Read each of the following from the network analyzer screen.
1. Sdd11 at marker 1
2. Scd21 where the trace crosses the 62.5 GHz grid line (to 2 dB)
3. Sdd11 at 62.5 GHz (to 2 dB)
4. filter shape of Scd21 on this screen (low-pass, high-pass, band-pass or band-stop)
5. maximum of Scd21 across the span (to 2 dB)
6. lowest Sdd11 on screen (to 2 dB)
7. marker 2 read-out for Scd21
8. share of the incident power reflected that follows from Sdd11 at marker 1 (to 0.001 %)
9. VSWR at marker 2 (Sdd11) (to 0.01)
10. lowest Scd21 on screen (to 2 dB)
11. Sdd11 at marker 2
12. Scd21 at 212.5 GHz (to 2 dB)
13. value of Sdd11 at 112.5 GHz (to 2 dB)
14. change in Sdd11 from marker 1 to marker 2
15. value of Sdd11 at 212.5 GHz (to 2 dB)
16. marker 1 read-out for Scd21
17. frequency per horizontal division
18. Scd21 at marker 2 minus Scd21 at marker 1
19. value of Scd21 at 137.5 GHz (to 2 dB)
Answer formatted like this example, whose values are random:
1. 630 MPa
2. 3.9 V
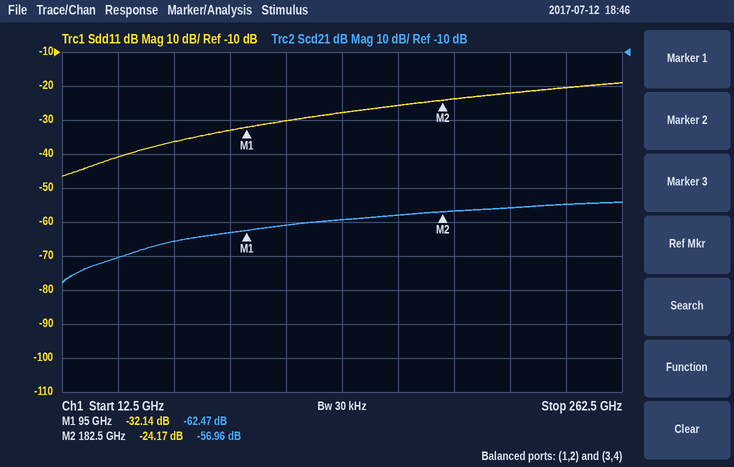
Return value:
1. -32.14 dB
2. -66 dB
3. -36 dB
4. high-pass
5. -54 dB
6. -46 dB
7. -56.96 dB
8. 0.061 %
9. 1.13
10. -78 dB
11. -24.17 dB
12. -56 dB
13. -30 dB
14. 7.97 dB
15. -22 dB
16. -62.47 dB
17. 25 GHz
18. 5.51 dB
19. -60 dB
